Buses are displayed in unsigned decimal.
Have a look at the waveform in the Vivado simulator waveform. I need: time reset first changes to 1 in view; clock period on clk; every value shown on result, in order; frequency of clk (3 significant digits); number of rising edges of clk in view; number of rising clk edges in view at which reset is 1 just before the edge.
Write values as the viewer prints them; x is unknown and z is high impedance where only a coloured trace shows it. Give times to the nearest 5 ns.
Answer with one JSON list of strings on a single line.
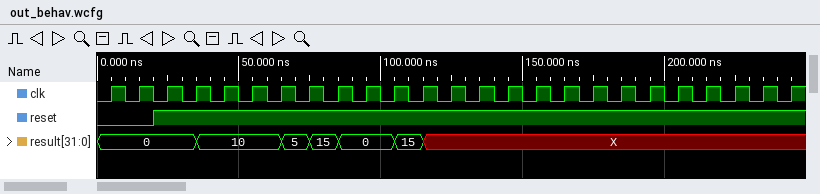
["20 ns", "10 ns", "0, 10, 5, 15, 0, 15, X", "100 MHz", "25", "23"]
